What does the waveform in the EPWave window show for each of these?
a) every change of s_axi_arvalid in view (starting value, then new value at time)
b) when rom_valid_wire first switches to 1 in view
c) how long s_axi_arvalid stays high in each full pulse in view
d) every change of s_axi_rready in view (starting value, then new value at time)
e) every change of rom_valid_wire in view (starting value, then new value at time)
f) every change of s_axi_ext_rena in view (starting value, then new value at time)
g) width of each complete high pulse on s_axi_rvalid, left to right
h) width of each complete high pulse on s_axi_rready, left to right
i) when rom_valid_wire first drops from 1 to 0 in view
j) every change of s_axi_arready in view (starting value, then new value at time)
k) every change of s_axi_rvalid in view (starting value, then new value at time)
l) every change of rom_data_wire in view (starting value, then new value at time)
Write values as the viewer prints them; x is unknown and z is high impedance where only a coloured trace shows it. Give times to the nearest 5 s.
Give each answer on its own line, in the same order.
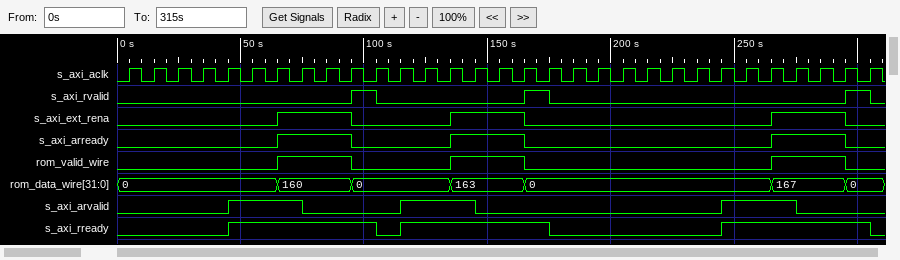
0, 1 at 45 s, 0 at 75 s, 1 at 115 s, 0 at 145 s, 1 at 245 s, 0 at 275 s
65 s
30 s, 30 s, 30 s
0, 1 at 45 s, 0 at 105 s, 1 at 115 s, 0 at 175 s, 1 at 245 s, 0 at 305 s
0, 1 at 65 s, 0 at 95 s, 1 at 135 s, 0 at 165 s, 1 at 265 s, 0 at 295 s
0, 1 at 65 s, 0 at 95 s, 1 at 135 s, 0 at 165 s, 1 at 265 s, 0 at 295 s
10 s, 10 s, 10 s
60 s, 60 s, 60 s
95 s
0, 1 at 65 s, 0 at 95 s, 1 at 135 s, 0 at 165 s, 1 at 265 s, 0 at 295 s
0, 1 at 95 s, 0 at 105 s, 1 at 165 s, 0 at 175 s, 1 at 295 s, 0 at 305 s
0, 160 at 65 s, 0 at 95 s, 163 at 135 s, 0 at 165 s, 167 at 265 s, 0 at 295 s
